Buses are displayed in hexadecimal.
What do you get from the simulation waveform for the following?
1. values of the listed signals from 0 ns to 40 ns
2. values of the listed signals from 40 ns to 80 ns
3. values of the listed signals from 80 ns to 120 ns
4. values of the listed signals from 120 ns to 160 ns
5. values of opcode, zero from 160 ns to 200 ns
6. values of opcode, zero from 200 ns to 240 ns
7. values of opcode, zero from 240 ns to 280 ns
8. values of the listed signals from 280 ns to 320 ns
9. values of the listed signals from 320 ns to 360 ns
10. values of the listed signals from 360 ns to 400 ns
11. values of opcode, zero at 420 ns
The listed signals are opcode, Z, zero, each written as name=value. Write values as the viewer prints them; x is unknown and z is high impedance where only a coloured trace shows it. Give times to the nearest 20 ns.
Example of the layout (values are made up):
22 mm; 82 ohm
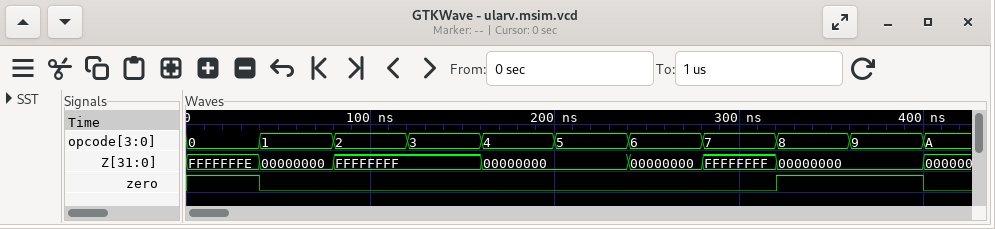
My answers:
opcode=0, Z=FFFFFFFE, zero=1; opcode=1, Z=00000000, zero=0; opcode=2, Z=FFFFFFFF, zero=0; opcode=3, Z=FFFFFFFF, zero=0; opcode=4, zero=0; opcode=5, zero=0; opcode=6, zero=0; opcode=7, Z=FFFFFFFF, zero=0; opcode=8, Z=00000000, zero=1; opcode=9, Z=00000000, zero=1; opcode=A, zero=0
